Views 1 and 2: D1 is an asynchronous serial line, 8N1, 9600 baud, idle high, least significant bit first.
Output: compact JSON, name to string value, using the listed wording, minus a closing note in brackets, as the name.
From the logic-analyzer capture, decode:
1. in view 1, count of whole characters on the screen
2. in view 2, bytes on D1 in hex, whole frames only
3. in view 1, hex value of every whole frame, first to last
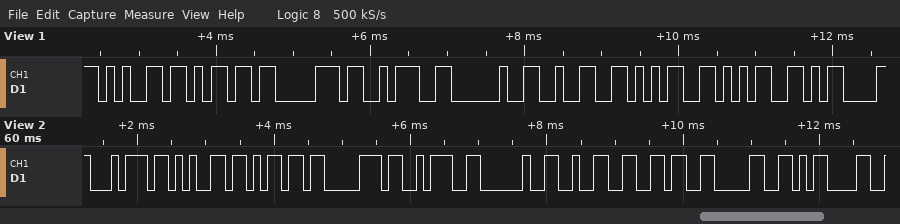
{"in view 1, count of whole characters on the screen": "9", "in view 2, bytes on D1 in hex, whole frames only": "0x74 0x65 0x6D 0x70 0x3A 0x20 0x32 0x36 0x30 0x0D", "in view 1, hex value of every whole frame, first to last": "65 6D 70 3A 20 32 35 35 0D"}
